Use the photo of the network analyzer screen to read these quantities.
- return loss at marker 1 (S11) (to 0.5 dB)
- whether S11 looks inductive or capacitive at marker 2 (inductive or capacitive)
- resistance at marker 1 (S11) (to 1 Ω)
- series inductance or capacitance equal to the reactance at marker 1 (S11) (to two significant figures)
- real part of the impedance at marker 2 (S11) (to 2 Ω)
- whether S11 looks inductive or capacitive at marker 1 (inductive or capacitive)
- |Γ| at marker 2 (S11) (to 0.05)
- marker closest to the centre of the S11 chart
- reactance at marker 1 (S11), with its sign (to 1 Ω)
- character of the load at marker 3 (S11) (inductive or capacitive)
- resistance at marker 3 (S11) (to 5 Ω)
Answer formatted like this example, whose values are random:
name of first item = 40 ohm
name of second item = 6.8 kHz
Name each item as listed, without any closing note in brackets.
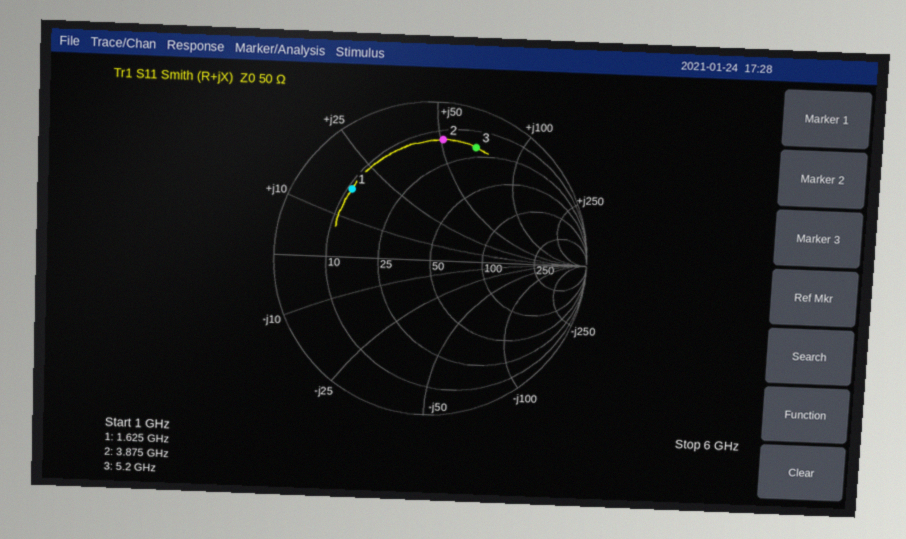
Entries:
return loss at marker 1 (S11) = 3.5 dB
whether S11 looks inductive or capacitive at marker 2 = inductive
resistance at marker 1 (S11) = 11 Ω
series inductance or capacitance equal to the reactance at marker 1 (S11) = 1.7 nH
real part of the impedance at marker 2 (S11) = 14 Ω
whether S11 looks inductive or capacitive at marker 1 = inductive
|Γ| at marker 2 (S11) = 0.75
marker closest to the centre of the S11 chart = marker 1
reactance at marker 1 (S11), with its sign = +17 Ω
character of the load at marker 3 (S11) = inductive
resistance at marker 3 (S11) = 20 Ω
